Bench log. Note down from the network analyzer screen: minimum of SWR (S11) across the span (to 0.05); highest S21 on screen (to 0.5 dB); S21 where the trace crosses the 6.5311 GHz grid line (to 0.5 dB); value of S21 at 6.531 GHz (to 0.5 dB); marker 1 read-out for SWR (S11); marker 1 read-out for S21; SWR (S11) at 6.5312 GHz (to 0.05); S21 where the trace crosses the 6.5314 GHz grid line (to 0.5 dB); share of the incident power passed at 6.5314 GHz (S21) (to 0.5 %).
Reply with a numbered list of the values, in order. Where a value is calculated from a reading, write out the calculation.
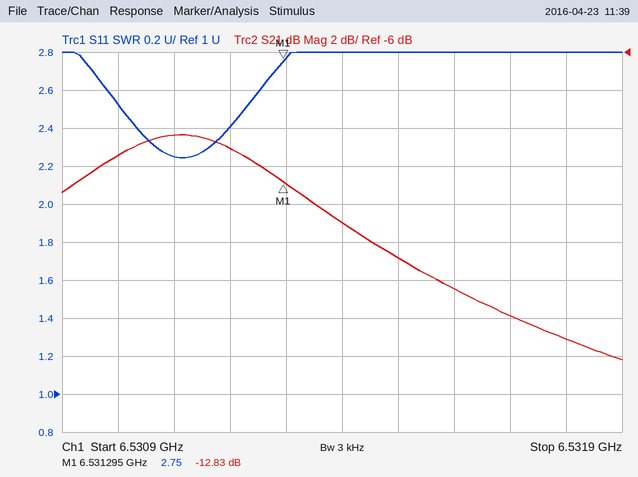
1. 2.25
2. -10.5 dB
3. -10.5 dB
4. -11.5 dB
5. 2.75
6. -12.83 dB
7. 2.40
8. -15.0 dB
9. 10^(-15/10) ≈ 3.16 %, so 3.0 % to the nearest 0.5 %
